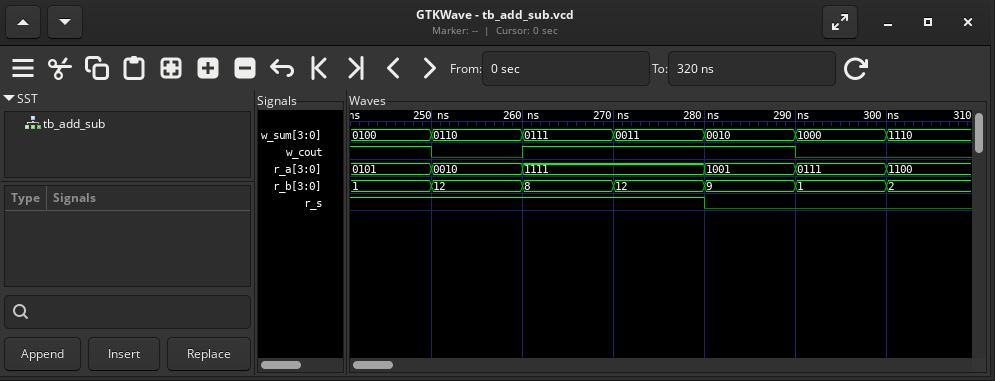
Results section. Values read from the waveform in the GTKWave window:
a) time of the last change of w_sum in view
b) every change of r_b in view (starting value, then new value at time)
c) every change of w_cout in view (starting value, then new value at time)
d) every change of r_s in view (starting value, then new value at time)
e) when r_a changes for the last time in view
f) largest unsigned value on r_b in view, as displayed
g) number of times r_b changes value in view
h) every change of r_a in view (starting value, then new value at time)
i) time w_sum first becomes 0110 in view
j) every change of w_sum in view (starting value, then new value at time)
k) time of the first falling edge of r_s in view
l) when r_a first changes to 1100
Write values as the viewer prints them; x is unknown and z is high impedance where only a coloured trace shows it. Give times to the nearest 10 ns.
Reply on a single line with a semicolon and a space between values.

300 ns; 1, 12 at 250 ns, 8 at 260 ns, 12 at 270 ns, 9 at 280 ns, 1 at 290 ns, 2 at 300 ns; 1, 0 at 250 ns, 1 at 260 ns, 0 at 290 ns; 1, 0 at 280 ns; 300 ns; 12; 6; 0101, 0010 at 250 ns, 1111 at 260 ns, 1001 at 280 ns, 0111 at 290 ns, 1100 at 300 ns; 250 ns; 0100, 0110 at 250 ns, 0111 at 260 ns, 0011 at 270 ns, 0010 at 280 ns, 1000 at 290 ns, 1110 at 300 ns; 280 ns; 300 ns
